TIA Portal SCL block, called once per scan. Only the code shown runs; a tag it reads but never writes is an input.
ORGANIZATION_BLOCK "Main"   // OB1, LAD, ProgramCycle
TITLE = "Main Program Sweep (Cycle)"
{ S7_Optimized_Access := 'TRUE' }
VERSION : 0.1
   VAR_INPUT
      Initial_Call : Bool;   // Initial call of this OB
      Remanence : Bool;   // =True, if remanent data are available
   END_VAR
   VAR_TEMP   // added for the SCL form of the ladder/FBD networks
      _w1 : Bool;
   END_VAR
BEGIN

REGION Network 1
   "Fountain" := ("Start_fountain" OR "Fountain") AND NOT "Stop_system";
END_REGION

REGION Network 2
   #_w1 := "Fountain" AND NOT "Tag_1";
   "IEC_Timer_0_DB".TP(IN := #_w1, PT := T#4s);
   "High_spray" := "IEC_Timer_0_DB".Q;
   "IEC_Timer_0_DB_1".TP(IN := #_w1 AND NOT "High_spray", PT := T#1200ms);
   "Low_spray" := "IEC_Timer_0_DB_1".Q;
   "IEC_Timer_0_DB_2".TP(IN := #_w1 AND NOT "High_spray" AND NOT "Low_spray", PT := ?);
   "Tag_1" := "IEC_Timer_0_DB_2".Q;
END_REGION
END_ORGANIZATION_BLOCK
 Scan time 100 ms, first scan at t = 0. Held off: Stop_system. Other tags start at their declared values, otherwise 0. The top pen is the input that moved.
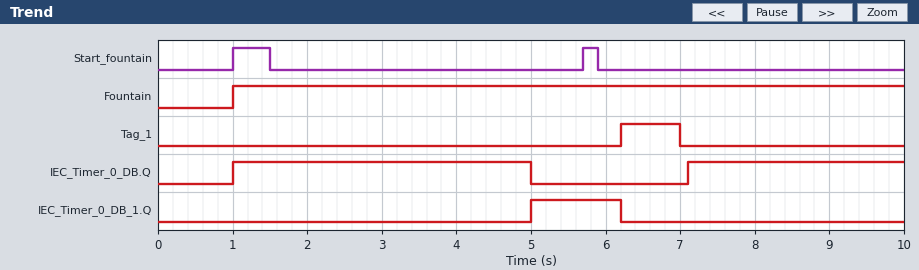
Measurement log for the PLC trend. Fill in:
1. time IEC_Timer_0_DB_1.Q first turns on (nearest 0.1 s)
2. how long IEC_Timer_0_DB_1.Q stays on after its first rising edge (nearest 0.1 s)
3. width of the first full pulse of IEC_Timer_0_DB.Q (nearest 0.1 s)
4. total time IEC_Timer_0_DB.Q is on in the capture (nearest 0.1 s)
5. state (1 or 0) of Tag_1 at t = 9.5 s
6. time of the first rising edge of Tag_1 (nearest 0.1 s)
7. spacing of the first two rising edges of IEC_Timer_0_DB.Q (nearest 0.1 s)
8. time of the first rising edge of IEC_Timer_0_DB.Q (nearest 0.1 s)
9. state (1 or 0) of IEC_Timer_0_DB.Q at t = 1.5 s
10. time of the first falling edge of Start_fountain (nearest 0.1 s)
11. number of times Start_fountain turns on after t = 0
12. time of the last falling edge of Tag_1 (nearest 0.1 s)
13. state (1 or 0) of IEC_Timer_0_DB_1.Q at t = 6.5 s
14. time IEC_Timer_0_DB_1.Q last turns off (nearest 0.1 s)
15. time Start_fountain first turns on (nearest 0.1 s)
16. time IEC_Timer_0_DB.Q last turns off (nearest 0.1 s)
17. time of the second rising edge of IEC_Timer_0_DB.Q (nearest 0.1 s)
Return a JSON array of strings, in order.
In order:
["5.0 s", "1.2 s", "4.0 s", "6.9 s", "0", "6.2 s", "6.1 s", "1.0 s", "1", "1.5 s", "2", "7.0 s", "0", "6.2 s", "1.0 s", "5.0 s", "7.1 s"]
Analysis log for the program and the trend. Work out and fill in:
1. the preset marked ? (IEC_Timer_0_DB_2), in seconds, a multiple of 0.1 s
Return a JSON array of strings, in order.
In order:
["0.8 s"]
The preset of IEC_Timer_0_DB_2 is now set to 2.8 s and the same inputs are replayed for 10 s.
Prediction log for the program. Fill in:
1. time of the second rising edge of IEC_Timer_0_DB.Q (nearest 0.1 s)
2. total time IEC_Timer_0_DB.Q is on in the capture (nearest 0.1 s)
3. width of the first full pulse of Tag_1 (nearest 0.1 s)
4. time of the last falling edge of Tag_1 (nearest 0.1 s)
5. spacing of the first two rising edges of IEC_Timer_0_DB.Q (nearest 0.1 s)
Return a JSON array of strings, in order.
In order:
["9.1 s", "4.9 s", "2.8 s", "9.0 s", "8.1 s"]
